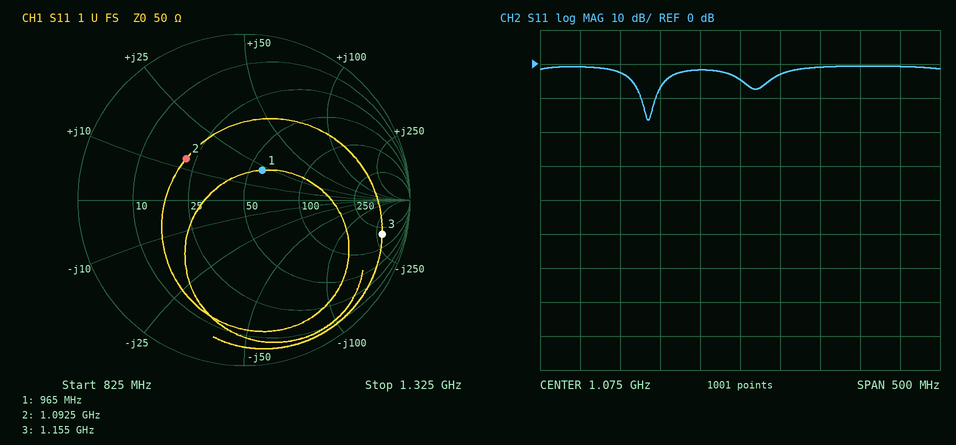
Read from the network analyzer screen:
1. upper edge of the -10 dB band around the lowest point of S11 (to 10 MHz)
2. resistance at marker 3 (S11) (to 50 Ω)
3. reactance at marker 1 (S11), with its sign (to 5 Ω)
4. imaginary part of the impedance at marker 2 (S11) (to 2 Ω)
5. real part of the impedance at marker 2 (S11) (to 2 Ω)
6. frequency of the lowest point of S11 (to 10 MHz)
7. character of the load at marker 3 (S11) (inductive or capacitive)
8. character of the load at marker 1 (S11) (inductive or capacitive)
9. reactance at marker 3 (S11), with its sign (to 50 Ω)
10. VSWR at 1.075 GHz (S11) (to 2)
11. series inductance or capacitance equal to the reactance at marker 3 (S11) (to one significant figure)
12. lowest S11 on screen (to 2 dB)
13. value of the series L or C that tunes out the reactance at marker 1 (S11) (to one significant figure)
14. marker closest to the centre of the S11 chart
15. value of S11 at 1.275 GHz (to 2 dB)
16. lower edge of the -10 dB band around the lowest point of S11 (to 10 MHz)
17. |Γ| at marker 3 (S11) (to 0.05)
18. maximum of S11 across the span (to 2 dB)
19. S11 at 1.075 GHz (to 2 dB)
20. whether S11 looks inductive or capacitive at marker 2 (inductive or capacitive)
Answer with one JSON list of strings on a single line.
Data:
["970 MHz", "200 Ω", "+20 Ω", "+14 Ω", "22 Ω", "960 MHz", "capacitive", "inductive", "-300 Ω", "4", "500 fF", "-16 dB", "8 pF", "marker 1", "0 dB", "950 MHz", "0.85", "0 dB", "-4 dB", "inductive"]
